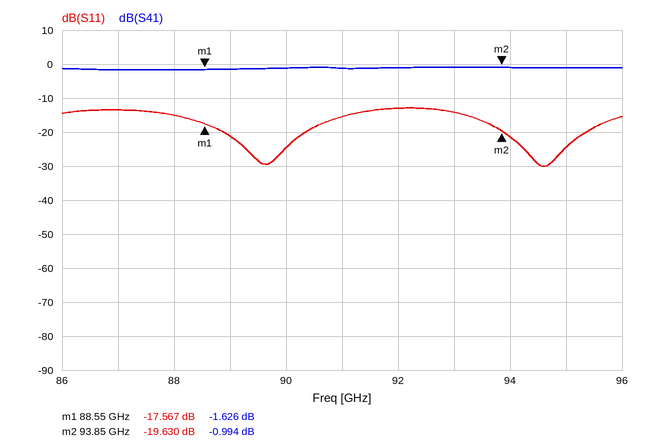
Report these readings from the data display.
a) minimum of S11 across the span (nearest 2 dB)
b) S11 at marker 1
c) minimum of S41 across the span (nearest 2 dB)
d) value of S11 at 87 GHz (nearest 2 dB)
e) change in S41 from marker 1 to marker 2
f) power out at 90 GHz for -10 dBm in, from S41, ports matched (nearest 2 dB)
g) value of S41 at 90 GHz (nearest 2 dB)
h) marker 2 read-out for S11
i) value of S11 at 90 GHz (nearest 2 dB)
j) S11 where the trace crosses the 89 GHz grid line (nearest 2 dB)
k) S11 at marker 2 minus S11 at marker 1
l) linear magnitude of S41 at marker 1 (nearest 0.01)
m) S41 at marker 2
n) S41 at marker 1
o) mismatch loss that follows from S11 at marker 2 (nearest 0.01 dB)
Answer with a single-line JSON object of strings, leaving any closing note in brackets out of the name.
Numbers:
{"minimum of S11 across the span": "-30 dB", "S11 at marker 1": "-17.567 dB", "minimum of S41 across the span": "-2 dB", "value of S11 at 87 GHz": "-14 dB", "change in S41 from marker 1 to marker 2": "0.632 dB", "power out at 90 GHz for -10 dBm in, from S41, ports matched": "-12 dBm", "value of S41 at 90 GHz": "-2 dB", "marker 2 read-out for S11": "-19.630 dB", "value of S11 at 90 GHz": "-24 dB", "S11 where the trace crosses the 89 GHz grid line": "-22 dB", "S11 at marker 2 minus S11 at marker 1": "-2.063 dB", "linear magnitude of S41 at marker 1": "0.83", "S41 at marker 2": "-0.994 dB", "S41 at marker 1": "-1.626 dB", "mismatch loss that follows from S11 at marker 2": "0.05 dB"}
